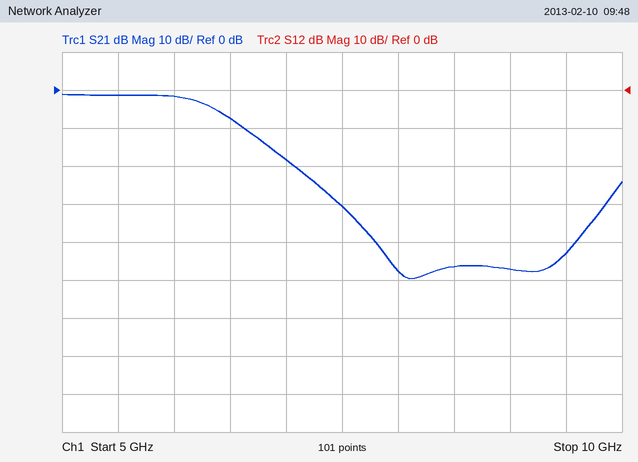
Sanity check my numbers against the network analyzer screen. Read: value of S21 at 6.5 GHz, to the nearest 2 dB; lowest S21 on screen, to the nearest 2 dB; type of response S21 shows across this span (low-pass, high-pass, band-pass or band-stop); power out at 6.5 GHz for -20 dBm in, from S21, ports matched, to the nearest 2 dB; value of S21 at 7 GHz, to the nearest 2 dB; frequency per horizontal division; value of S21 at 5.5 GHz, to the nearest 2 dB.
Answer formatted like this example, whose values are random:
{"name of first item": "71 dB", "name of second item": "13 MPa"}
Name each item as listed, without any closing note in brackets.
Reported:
{"value of S21 at 6.5 GHz, to the nearest 2 dB": "-8 dB", "lowest S21 on screen, to the nearest 2 dB": "-50 dB", "type of response S21 shows across this span": "low-pass", "power out at 6.5 GHz for -20 dBm in, from S21, ports matched, to the nearest 2 dB": "-28 dBm", "value of S21 at 7 GHz, to the nearest 2 dB": "-18 dB", "frequency per horizontal division": "500 MHz", "value of S21 at 5.5 GHz, to the nearest 2 dB": "-2 dB"}
